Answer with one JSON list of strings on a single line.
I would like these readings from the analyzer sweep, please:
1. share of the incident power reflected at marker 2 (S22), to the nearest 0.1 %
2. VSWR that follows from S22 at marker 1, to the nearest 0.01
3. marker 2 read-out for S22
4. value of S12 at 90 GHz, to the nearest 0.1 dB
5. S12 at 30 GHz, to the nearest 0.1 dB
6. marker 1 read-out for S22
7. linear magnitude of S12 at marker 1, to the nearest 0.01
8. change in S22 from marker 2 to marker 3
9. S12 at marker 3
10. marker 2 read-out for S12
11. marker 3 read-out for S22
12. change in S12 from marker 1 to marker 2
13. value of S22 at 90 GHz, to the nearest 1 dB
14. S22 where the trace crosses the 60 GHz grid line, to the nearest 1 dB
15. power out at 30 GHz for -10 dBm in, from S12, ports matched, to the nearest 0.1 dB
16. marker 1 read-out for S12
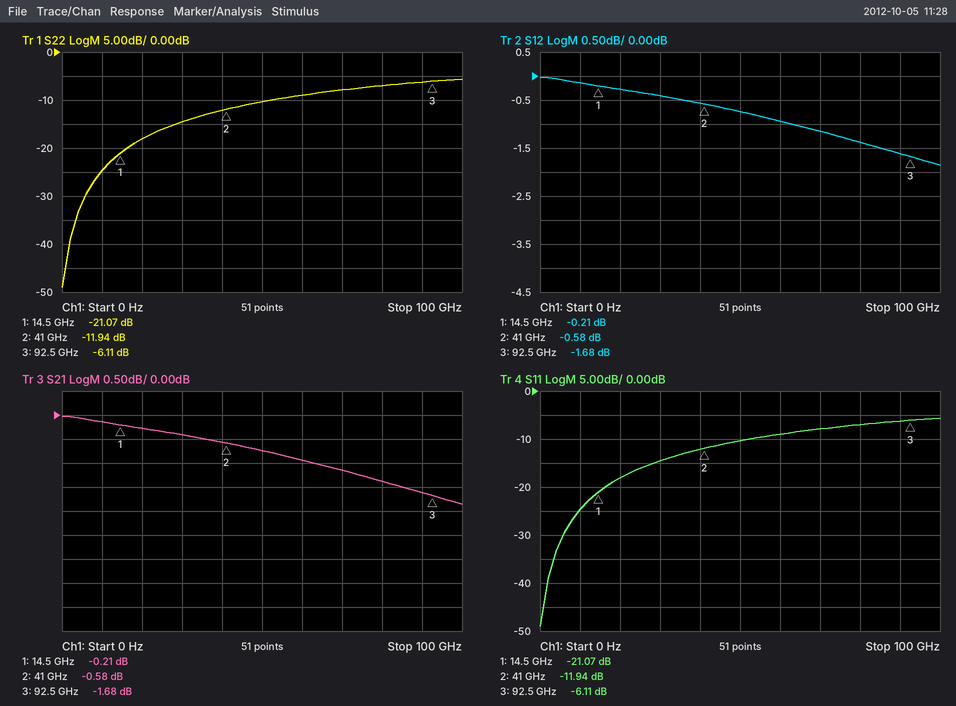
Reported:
["6.4 %", "1.19", "-11.94 dB", "-1.6 dB", "-0.4 dB", "-21.07 dB", "0.98", "5.83 dB", "-1.68 dB", "-0.58 dB", "-6.11 dB", "-0.37 dB", "-6 dB", "-9 dB", "-10.4 dBm", "-0.21 dB"]
